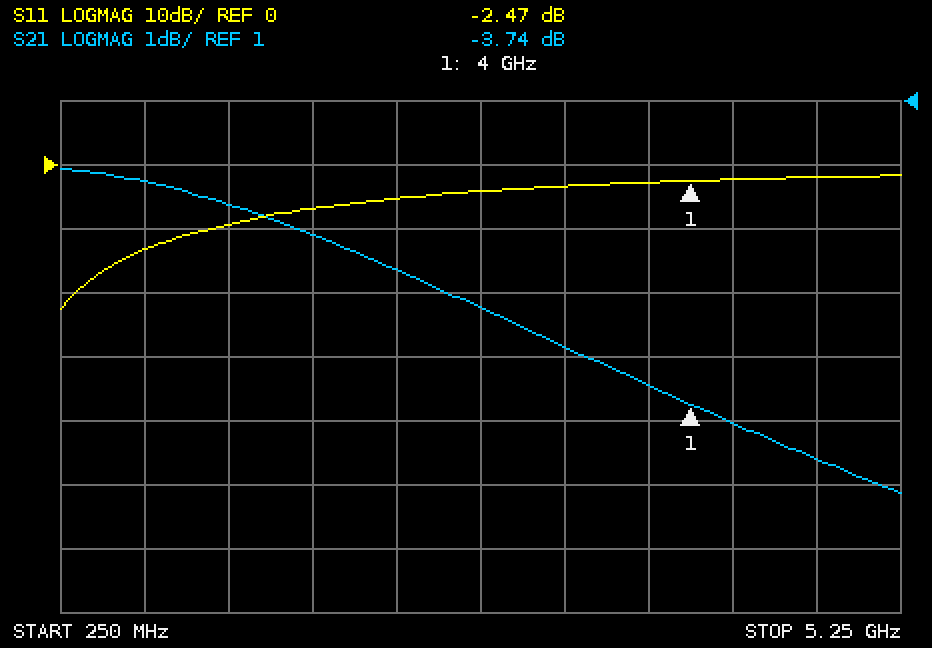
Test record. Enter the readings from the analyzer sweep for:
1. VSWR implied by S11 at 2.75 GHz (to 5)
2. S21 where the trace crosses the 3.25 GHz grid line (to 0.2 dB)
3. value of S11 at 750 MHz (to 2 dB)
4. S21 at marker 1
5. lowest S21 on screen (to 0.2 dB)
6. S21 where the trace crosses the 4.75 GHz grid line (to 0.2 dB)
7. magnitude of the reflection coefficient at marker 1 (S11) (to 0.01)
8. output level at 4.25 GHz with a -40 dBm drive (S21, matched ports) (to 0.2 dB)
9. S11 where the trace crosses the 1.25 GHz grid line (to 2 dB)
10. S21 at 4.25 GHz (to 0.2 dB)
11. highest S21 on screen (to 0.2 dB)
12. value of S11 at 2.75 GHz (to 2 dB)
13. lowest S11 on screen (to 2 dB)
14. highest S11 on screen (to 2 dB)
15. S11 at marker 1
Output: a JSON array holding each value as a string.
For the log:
["5", "-2.8 dB", "-14 dB", "-3.74 dB", "-5.2 dB", "-4.6 dB", "0.75", "-44.0 dBm", "-10 dB", "-4.0 dB", "0.0 dB", "-4 dB", "-22 dB", "-2 dB", "-2.47 dB"]
